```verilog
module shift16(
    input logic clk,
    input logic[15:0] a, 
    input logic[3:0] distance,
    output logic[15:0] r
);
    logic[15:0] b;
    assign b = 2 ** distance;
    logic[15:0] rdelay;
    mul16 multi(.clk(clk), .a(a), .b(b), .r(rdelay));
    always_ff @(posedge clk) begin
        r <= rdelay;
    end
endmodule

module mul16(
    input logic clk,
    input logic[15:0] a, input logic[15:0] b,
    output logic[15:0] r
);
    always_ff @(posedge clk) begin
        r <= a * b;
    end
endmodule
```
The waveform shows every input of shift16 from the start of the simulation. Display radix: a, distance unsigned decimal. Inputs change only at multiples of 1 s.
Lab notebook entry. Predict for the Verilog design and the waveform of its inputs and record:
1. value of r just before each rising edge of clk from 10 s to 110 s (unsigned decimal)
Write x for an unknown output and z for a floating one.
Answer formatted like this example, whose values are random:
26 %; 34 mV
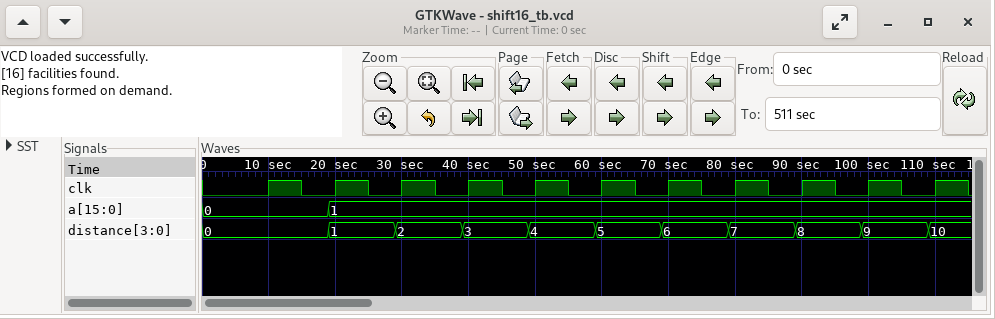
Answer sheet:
x, x, 0, 2, 4, 8, 16, 32, 64, 128, 256
